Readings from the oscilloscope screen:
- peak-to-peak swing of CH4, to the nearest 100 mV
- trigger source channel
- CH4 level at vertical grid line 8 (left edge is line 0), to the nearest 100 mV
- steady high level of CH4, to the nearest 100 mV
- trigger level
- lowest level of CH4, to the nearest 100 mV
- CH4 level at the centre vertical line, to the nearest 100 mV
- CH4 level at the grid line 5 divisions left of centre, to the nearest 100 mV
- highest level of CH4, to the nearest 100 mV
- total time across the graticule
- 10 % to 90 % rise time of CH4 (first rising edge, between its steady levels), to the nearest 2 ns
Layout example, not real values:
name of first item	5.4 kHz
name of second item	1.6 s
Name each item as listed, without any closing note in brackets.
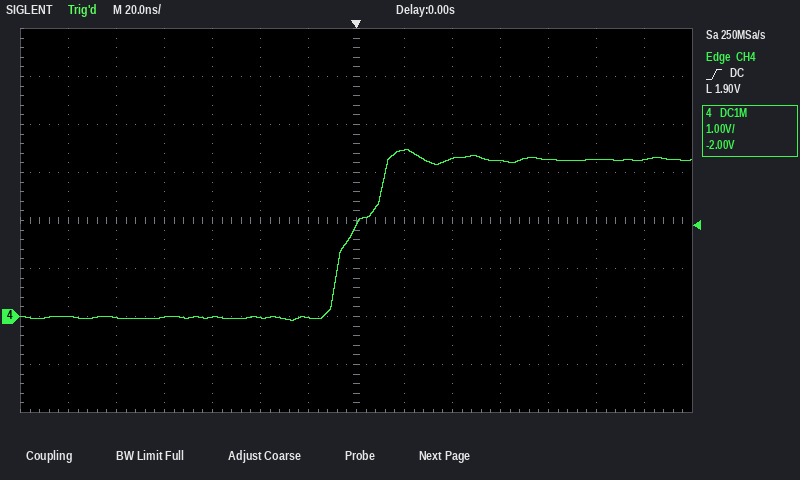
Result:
peak-to-peak swing of CH4, to the nearest 100 mV	3.6 V
trigger source channel	CH4
CH4 level at vertical grid line 8 (left edge is line 0), to the nearest 100 mV	3.5 V
steady high level of CH4, to the nearest 100 mV	3.3 V
trigger level	1.90 V
lowest level of CH4, to the nearest 100 mV	-100 mV
CH4 level at the centre vertical line, to the nearest 100 mV	1.9 V
CH4 level at the grid line 5 divisions left of centre, to the nearest 100 mV	0.0 V
highest level of CH4, to the nearest 100 mV	3.5 V
total time across the graticule	280 ns
10 % to 90 % rise time of CH4 (first rising edge, between its steady levels), to the nearest 2 ns	22 ns
